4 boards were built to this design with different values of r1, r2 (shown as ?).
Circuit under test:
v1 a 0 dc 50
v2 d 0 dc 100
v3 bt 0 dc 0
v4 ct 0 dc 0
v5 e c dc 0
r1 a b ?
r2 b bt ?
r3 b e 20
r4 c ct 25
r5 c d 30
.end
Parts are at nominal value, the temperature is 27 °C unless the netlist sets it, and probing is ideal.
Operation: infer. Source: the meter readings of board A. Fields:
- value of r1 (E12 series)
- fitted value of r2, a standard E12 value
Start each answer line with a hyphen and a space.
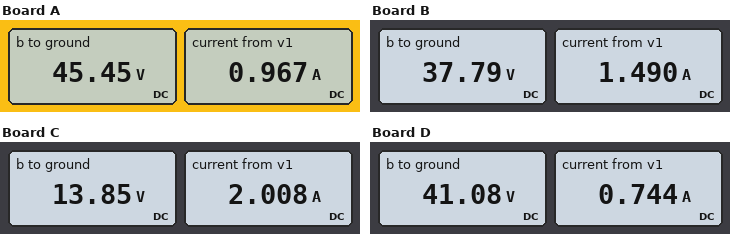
- 4.7 Ω
- 47 Ω
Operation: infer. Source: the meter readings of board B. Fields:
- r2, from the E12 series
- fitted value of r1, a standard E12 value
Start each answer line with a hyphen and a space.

- 22 Ω
- 8.2 Ω
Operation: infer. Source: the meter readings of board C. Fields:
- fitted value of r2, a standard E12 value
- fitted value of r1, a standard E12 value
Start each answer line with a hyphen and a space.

- 4.7 Ω
- 18 Ω
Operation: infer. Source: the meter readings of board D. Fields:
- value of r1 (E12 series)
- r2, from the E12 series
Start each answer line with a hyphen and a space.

- 12 Ω
- 47 Ω
